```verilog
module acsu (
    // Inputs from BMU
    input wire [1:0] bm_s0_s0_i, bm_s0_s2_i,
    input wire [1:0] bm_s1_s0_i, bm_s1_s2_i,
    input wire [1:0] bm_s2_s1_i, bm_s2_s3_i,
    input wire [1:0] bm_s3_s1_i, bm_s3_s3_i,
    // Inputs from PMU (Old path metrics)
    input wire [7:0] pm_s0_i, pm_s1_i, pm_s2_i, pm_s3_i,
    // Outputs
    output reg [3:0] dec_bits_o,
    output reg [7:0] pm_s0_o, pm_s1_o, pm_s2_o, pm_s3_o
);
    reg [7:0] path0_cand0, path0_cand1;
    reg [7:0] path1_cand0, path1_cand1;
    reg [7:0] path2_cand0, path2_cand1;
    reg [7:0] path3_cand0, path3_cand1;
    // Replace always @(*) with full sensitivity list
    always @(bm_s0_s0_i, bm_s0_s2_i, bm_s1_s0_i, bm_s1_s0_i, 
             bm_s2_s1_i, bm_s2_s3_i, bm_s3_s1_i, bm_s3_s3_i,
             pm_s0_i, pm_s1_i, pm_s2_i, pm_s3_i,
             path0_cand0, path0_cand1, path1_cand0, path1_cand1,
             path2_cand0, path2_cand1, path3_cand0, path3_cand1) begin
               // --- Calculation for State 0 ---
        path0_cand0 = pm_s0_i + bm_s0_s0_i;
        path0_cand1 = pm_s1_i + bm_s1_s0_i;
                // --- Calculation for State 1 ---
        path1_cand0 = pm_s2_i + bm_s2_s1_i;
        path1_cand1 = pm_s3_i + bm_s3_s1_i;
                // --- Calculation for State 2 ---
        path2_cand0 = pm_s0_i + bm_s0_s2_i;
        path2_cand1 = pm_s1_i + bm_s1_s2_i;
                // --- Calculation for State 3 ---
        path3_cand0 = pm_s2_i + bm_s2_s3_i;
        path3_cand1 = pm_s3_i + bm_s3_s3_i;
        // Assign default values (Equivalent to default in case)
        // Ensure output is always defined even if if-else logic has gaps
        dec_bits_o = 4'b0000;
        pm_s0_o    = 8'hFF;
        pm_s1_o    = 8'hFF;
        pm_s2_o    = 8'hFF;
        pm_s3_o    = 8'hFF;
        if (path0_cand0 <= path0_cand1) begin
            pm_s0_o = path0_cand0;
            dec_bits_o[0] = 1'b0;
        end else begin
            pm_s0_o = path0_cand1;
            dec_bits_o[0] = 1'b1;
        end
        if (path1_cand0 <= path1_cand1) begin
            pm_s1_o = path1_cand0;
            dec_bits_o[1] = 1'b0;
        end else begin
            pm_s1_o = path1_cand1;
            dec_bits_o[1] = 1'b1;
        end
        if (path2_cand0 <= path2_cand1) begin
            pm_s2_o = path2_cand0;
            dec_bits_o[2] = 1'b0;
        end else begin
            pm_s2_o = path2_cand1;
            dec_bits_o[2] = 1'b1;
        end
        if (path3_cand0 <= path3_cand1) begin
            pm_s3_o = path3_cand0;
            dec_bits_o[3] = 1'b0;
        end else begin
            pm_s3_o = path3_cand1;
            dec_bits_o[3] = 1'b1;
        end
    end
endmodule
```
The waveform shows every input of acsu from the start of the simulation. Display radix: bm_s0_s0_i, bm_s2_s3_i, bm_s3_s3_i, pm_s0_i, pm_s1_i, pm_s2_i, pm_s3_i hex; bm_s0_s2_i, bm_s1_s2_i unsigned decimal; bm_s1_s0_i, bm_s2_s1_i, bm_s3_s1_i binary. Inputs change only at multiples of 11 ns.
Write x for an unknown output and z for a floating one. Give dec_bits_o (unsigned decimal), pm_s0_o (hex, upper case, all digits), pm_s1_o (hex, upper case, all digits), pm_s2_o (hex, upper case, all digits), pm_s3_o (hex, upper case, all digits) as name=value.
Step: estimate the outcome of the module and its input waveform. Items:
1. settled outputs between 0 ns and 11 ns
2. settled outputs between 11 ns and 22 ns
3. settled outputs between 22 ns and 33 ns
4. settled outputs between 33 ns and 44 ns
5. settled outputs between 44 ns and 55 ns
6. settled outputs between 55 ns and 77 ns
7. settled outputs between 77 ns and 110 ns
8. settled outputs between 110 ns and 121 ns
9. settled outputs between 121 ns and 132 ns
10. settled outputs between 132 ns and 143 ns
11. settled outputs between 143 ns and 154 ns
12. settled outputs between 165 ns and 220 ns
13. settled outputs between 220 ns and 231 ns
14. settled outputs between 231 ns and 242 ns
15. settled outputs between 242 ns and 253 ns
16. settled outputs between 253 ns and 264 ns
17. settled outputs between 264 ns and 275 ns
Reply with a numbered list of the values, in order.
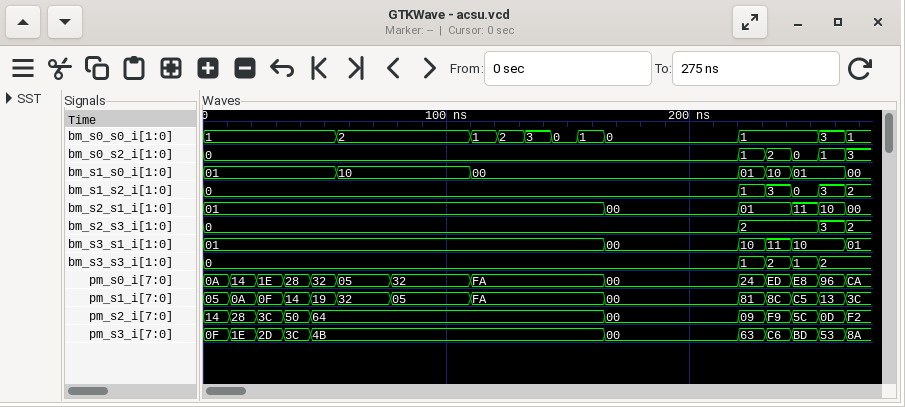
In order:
1. dec_bits_o=15, pm_s0_o=06, pm_s1_o=10, pm_s2_o=05, pm_s3_o=0F
2. dec_bits_o=15, pm_s0_o=0B, pm_s1_o=1F, pm_s2_o=0A, pm_s3_o=1E
3. dec_bits_o=15, pm_s0_o=10, pm_s1_o=2E, pm_s2_o=0F, pm_s3_o=2D
4. dec_bits_o=15, pm_s0_o=15, pm_s1_o=3D, pm_s2_o=14, pm_s3_o=3C
5. dec_bits_o=15, pm_s0_o=1A, pm_s1_o=4C, pm_s2_o=19, pm_s3_o=4B
6. dec_bits_o=10, pm_s0_o=07, pm_s1_o=4C, pm_s2_o=05, pm_s3_o=4B
7. dec_bits_o=15, pm_s0_o=07, pm_s1_o=4C, pm_s2_o=05, pm_s3_o=4B
8. dec_bits_o=11, pm_s0_o=FA, pm_s1_o=4C, pm_s2_o=FA, pm_s3_o=4B
9. dec_bits_o=11, pm_s0_o=FA, pm_s1_o=4C, pm_s2_o=FA, pm_s3_o=4B
10. dec_bits_o=11, pm_s0_o=FA, pm_s1_o=4C, pm_s2_o=FA, pm_s3_o=4B
11. dec_bits_o=10, pm_s0_o=FA, pm_s1_o=4C, pm_s2_o=FA, pm_s3_o=4B
12. dec_bits_o=0, pm_s0_o=00, pm_s1_o=00, pm_s2_o=00, pm_s3_o=00
13. dec_bits_o=0, pm_s0_o=25, pm_s1_o=0A, pm_s2_o=25, pm_s3_o=0B
14. dec_bits_o=15, pm_s0_o=8E, pm_s1_o=C9, pm_s2_o=8F, pm_s3_o=C8
15. dec_bits_o=5, pm_s0_o=C6, pm_s1_o=5F, pm_s2_o=C5, pm_s3_o=5E
16. dec_bits_o=5, pm_s0_o=14, pm_s1_o=0F, pm_s2_o=16, pm_s3_o=10
17. dec_bits_o=15, pm_s0_o=3C, pm_s1_o=8B, pm_s2_o=3E, pm_s3_o=8C
